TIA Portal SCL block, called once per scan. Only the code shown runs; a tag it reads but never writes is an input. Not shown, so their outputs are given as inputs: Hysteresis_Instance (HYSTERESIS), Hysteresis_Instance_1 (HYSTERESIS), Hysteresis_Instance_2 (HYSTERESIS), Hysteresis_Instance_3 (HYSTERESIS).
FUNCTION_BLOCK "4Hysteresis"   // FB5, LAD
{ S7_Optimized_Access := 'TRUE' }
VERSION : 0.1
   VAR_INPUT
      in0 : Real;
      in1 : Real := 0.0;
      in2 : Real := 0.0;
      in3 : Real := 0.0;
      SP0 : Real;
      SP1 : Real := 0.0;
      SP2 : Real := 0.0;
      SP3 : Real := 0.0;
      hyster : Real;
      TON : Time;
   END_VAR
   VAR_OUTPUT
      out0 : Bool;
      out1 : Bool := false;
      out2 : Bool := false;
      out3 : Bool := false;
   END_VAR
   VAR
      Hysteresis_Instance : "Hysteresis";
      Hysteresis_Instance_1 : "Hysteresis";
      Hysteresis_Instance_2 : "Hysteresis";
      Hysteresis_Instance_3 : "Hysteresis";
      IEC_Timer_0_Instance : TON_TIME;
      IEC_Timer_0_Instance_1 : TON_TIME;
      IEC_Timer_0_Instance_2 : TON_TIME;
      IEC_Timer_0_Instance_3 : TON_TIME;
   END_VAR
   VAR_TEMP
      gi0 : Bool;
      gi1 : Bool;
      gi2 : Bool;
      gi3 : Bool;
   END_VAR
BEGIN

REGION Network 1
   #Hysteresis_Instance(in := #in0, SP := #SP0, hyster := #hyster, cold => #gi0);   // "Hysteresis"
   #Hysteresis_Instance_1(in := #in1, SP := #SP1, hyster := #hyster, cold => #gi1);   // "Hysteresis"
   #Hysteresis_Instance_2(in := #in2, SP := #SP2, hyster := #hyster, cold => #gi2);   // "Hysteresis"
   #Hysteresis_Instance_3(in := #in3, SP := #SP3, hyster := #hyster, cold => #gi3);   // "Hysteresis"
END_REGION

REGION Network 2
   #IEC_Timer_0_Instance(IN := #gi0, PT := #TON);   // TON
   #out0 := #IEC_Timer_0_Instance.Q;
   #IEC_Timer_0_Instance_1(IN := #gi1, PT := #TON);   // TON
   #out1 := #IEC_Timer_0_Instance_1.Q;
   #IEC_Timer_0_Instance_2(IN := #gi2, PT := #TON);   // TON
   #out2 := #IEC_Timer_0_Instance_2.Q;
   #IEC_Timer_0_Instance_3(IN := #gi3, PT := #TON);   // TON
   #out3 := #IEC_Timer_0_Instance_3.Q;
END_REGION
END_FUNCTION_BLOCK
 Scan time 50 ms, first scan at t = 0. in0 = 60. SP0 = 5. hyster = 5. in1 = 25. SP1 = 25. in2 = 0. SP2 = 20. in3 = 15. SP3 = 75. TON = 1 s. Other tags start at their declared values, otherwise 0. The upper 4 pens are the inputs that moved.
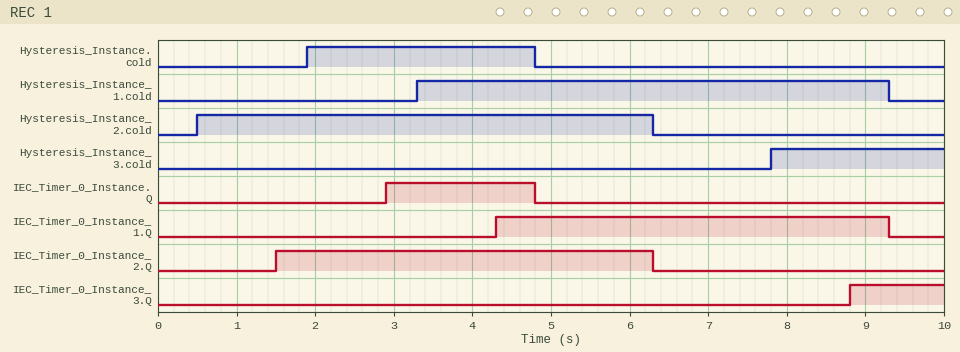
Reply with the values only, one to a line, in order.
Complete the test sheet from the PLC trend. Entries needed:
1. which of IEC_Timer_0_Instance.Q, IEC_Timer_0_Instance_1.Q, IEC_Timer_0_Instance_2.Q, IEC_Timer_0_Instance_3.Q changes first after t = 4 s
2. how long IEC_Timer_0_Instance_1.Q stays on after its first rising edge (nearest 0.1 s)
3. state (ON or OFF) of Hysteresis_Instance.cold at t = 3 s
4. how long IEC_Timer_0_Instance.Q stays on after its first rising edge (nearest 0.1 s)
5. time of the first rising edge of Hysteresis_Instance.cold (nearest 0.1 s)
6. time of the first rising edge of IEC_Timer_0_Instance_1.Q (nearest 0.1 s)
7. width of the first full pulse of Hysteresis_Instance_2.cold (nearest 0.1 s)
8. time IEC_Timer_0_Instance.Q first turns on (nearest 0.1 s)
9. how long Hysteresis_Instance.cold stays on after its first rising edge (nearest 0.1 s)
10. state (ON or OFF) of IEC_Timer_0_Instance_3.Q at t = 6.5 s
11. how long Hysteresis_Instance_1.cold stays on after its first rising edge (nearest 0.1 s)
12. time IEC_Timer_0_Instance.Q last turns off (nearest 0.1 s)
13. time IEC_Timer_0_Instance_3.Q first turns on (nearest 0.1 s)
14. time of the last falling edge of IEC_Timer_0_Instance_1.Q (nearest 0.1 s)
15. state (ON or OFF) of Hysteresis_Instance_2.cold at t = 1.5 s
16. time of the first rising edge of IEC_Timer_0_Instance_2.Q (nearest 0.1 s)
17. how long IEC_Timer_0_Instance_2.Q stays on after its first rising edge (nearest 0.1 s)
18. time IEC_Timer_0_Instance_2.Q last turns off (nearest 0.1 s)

IEC_Timer_0_Instance_1.Q
5.0 s
ON
1.9 s
1.9 s
4.3 s
5.8 s
2.9 s
2.9 s
OFF
6.0 s
4.8 s
8.8 s
9.3 s
ON
1.5 s
4.8 s
6.3 s
